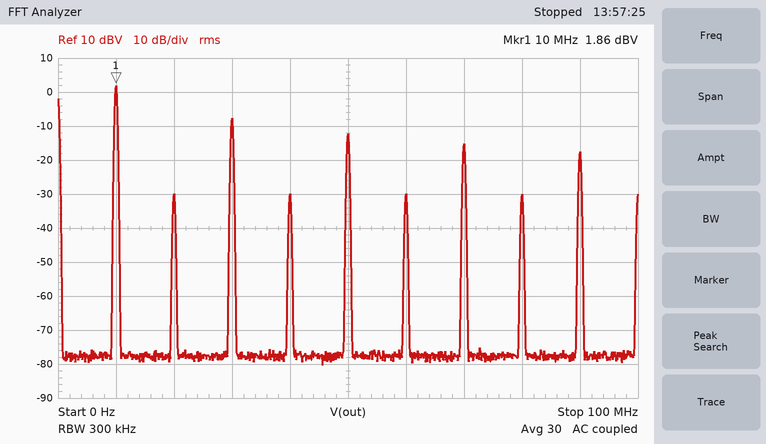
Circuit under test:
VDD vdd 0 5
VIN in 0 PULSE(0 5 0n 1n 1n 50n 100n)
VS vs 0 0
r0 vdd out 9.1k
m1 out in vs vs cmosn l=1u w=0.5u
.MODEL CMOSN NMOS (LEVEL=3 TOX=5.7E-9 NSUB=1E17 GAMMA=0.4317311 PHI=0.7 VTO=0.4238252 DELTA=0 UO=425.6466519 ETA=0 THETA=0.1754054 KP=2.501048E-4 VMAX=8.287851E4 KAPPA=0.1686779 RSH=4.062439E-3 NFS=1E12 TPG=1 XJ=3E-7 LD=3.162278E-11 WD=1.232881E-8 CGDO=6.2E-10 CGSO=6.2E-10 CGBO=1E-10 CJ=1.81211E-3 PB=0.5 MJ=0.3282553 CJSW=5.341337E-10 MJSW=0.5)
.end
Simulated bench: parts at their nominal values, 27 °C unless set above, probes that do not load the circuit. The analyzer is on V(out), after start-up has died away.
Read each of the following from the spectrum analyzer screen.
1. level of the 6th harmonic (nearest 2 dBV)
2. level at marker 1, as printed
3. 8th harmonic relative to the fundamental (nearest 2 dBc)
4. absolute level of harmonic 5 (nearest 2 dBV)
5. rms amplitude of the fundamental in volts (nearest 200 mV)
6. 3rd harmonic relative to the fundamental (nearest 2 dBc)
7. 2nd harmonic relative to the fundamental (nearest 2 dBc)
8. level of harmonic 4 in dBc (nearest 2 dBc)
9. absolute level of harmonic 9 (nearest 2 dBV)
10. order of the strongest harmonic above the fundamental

-30 dBV
1.86 dBV
-32 dBc
-12 dBV
1.2 V
-10 dBc
-32 dBc
-32 dBc
-18 dBV
3
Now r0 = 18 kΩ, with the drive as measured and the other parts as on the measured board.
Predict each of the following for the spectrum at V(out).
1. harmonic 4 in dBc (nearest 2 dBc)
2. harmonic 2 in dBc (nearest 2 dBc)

-30 dBc
-30 dBc
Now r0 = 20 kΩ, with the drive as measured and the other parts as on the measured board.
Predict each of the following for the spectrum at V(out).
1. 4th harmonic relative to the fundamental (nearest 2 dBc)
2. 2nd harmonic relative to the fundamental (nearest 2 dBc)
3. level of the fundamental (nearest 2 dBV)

-30 dBc
-30 dBc
6 dBV
